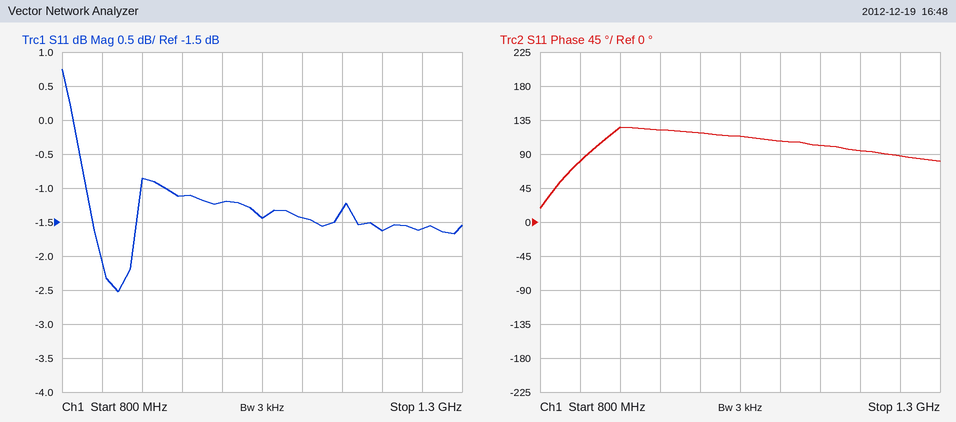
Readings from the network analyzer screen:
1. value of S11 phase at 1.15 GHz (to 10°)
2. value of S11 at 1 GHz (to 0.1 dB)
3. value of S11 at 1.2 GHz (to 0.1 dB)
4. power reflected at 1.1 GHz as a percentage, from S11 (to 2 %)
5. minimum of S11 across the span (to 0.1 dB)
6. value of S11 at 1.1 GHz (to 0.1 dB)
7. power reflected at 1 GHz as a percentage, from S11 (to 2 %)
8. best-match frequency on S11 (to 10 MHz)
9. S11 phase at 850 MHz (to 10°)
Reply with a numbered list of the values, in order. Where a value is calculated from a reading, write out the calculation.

1. 100°
2. -1.2 dB
3. -1.6 dB
4. 10^(-1.4/10) ≈ 72 %
5. -2.5 dB
6. -1.4 dB
7. 10^(-1.2/10) ≈ 76 %
8. 870 MHz
9. 80°
